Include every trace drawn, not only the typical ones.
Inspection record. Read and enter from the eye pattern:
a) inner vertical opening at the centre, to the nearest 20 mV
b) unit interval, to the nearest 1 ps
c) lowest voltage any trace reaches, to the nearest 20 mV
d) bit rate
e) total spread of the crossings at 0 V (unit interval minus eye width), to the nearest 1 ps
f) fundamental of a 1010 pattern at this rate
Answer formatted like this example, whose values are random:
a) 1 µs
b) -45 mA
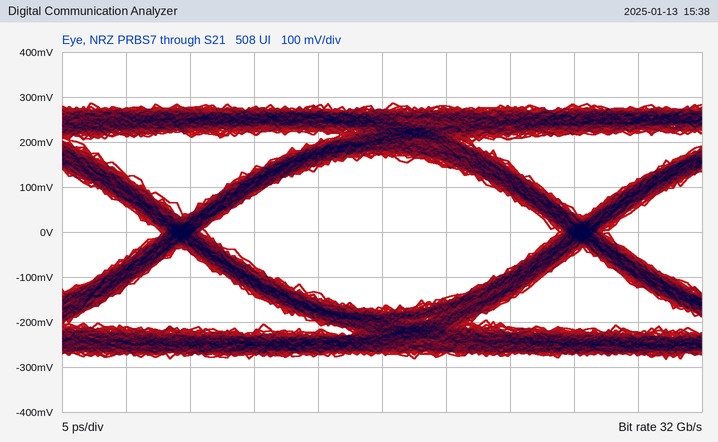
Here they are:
a) 340 mV
b) 31 ps
c) -280 mV
d) 32 Gb/s
e) 4 ps
f) 16 GHz
